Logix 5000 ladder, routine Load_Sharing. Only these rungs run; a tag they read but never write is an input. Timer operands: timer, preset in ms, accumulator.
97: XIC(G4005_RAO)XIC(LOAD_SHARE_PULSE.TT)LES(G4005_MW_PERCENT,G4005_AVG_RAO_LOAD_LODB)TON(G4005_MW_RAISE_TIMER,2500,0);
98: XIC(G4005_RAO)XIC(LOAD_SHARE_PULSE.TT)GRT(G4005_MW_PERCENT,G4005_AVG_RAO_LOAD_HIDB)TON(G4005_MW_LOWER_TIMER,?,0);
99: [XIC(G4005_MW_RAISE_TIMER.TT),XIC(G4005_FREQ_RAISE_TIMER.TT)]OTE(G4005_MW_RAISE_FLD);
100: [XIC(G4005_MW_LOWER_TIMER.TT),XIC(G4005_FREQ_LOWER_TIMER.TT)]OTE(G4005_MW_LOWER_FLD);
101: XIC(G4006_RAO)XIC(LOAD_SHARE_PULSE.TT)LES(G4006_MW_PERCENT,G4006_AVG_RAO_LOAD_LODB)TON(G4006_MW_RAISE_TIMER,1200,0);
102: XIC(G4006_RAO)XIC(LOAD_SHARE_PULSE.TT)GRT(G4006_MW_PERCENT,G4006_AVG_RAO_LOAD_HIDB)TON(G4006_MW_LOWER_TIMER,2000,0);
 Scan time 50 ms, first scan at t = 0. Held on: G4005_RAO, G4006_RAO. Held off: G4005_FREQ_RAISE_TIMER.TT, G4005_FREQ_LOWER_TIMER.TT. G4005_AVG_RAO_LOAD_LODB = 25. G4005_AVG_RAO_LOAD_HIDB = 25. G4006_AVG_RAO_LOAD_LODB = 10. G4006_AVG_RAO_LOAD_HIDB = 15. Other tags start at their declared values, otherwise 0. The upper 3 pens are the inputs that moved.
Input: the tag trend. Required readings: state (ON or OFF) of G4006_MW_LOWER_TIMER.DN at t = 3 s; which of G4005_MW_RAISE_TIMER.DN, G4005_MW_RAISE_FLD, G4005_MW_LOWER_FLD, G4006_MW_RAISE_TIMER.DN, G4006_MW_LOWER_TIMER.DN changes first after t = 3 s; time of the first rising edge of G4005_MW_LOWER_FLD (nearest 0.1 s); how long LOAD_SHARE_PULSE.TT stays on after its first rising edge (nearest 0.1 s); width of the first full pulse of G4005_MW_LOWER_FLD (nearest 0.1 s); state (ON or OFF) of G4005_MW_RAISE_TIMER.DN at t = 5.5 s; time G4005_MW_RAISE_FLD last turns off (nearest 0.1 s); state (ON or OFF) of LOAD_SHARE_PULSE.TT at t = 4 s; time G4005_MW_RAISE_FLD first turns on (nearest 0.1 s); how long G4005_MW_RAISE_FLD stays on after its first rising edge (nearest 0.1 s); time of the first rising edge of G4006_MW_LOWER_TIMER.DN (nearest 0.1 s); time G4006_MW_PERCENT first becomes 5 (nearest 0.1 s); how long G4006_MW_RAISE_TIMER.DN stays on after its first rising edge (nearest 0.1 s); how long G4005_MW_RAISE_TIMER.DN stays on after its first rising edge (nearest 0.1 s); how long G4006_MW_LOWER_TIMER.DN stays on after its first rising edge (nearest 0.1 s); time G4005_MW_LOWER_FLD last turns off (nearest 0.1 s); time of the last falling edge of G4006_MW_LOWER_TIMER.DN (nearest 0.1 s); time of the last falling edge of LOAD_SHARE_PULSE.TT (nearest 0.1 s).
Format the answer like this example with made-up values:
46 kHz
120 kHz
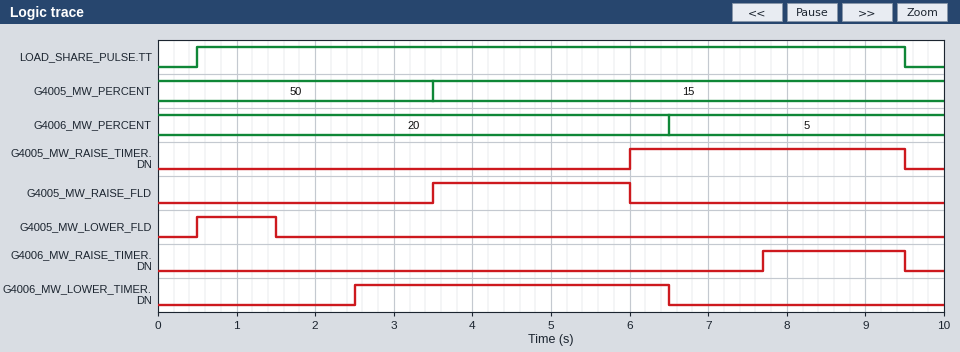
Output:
ON
G4005_MW_RAISE_FLD
0.5 s
9.0 s
1.0 s
OFF
6.0 s
ON
3.5 s
2.5 s
2.5 s
6.5 s
1.8 s
3.5 s
4.0 s
1.5 s
6.5 s
9.5 s
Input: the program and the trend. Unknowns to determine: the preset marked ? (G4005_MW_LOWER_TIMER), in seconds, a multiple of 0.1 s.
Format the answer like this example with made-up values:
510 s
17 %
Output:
1.0 s
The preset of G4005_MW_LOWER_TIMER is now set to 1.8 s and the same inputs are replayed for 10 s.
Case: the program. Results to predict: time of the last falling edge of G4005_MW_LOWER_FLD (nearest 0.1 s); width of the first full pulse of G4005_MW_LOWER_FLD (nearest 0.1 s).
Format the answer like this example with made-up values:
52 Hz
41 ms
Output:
2.3 s
1.8 s
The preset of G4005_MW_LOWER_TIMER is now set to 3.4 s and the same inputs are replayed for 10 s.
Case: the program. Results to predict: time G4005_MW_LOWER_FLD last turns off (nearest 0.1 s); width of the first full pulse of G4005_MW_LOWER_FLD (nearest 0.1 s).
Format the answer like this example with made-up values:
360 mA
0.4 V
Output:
3.5 s
3.0 s
